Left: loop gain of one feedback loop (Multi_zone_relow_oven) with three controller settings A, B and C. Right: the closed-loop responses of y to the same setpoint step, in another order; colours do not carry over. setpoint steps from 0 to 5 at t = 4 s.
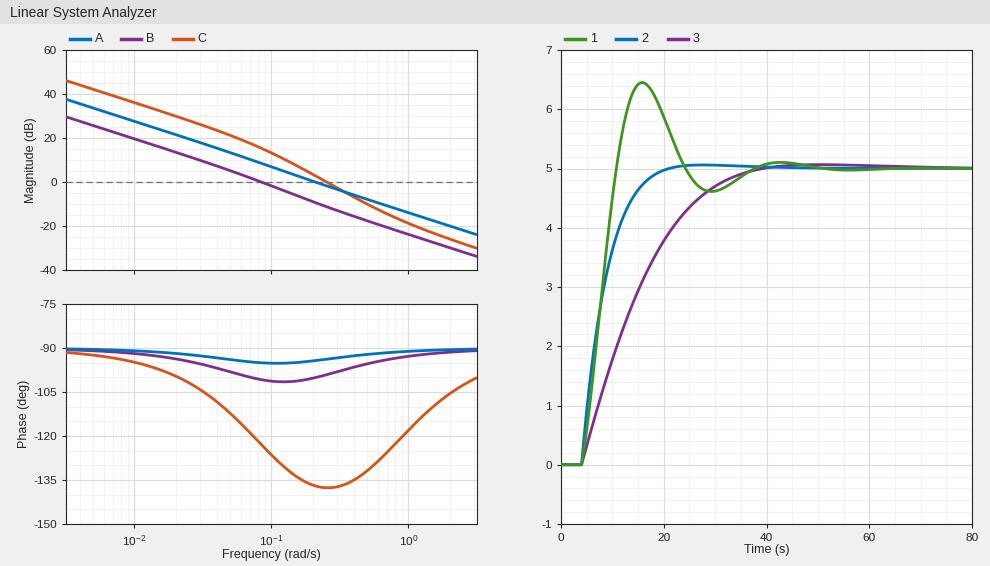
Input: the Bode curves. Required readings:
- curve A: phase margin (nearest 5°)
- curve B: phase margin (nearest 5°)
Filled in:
85°
80°
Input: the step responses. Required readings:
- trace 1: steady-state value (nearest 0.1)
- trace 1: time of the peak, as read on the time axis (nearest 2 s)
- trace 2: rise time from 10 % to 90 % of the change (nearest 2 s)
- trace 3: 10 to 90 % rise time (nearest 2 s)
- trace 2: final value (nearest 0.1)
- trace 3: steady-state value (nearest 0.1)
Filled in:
5.0
16 s
10 s
22 s
5.0
5.0
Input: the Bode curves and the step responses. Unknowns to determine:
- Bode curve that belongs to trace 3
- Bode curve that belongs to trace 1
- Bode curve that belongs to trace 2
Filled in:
B
C
A
